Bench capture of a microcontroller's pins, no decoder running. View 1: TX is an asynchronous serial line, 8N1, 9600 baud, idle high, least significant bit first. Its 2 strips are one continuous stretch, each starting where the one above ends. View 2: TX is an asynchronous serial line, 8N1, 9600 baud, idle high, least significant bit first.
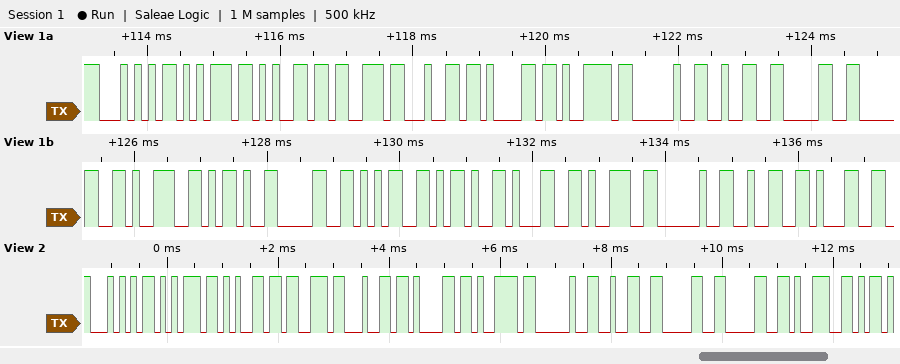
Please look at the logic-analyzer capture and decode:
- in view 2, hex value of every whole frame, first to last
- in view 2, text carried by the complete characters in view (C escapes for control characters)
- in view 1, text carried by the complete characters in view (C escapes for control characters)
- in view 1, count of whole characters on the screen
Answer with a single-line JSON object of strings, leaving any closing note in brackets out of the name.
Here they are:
{"in view 2, hex value of every whole frame, first to last": "54 75 65 73 64 61 79 20 32 30 30 39", "in view 2, text carried by the complete characters in view": "\"Tuesday 2009\"", "in view 1, text carried by the complete characters in view": "\"Tuesday 2009-05-19 21\"", "in view 1, count of whole characters on the screen": "21"}
